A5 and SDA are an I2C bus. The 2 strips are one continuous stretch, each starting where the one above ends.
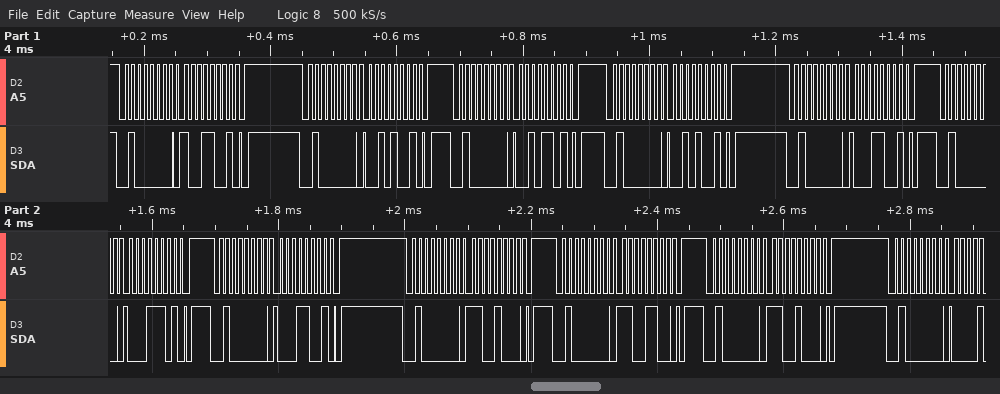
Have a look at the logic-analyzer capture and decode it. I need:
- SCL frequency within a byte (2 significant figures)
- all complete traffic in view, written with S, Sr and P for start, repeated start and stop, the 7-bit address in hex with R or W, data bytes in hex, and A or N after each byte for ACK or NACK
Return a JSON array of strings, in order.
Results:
["100 kHz", "S 20W A 99 A P S 20W A 29 A P S 20W A 2D A P S 20W A 29 A P S 20W A 19 A P S 20W A 1D A P S 20W A 19 A P S 20W A C8 A P S 20W A CC A P S 20W A C8 A P S 20W A"]
